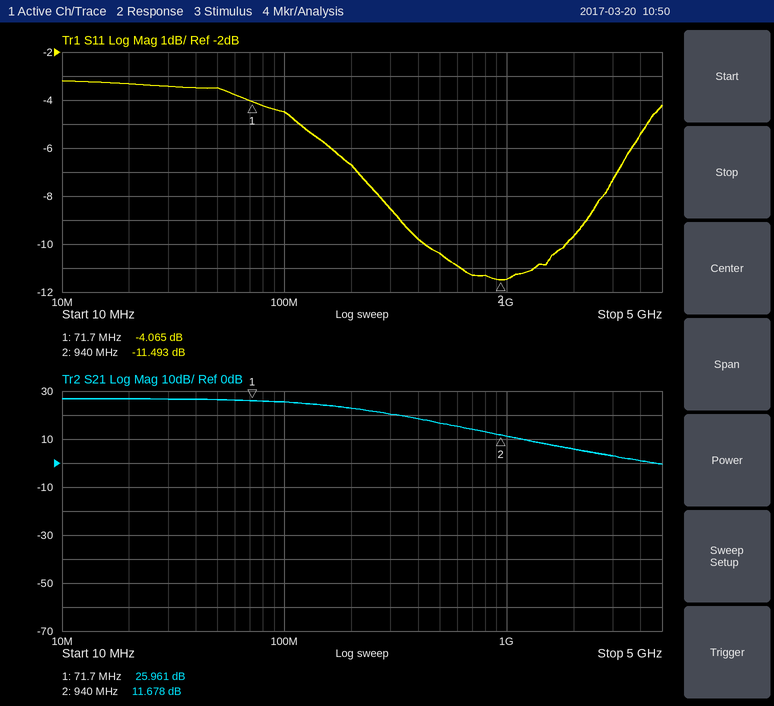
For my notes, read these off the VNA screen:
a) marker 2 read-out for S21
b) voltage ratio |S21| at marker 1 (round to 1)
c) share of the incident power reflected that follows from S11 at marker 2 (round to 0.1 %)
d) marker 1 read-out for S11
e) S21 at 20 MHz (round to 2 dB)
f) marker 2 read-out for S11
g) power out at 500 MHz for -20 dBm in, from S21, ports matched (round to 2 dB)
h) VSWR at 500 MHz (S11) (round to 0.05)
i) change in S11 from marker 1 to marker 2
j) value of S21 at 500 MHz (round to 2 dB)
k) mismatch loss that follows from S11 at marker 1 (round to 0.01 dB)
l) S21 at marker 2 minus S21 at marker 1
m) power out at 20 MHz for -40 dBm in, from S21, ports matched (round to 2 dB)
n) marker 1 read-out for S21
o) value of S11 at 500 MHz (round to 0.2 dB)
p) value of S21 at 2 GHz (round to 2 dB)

11.678 dB
20
7.1 %
-4.065 dB
26 dB
-11.493 dB
-4 dBm
1.85
-7.428 dB
16 dB
2.16 dB
-14.283 dB
-14 dBm
25.961 dB
-10.4 dB
6 dB
